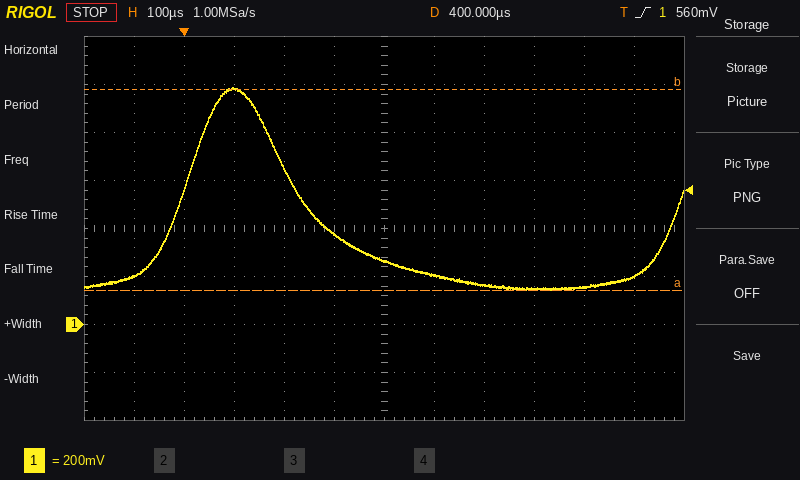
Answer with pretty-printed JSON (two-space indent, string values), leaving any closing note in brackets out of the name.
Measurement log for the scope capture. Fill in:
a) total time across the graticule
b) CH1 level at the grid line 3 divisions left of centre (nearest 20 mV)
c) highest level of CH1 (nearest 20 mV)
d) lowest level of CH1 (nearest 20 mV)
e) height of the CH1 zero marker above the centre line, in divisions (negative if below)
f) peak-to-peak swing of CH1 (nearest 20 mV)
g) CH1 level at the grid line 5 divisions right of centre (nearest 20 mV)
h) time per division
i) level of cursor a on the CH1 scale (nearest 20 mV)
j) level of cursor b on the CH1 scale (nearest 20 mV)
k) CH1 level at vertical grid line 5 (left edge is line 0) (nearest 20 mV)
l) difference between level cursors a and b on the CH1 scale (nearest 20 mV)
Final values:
{
  "total time across the graticule": "1.2 ms",
  "CH1 level at the grid line 3 divisions left of centre": "980 mV",
  "highest level of CH1": "980 mV",
  "lowest level of CH1": "140 mV",
  "height of the CH1 zero marker above the centre line, in divisions": "-2.0 div",
  "peak-to-peak swing of CH1": "840 mV",
  "CH1 level at the grid line 5 divisions right of centre": "200 mV",
  "time per division": "100 µs",
  "level of cursor a on the CH1 scale": "140 mV",
  "level of cursor b on the CH1 scale": "980 mV",
  "CH1 level at vertical grid line 5 (left edge is line 0)": "380 mV",
  "difference between level cursors a and b on the CH1 scale": "840 mV"
}
